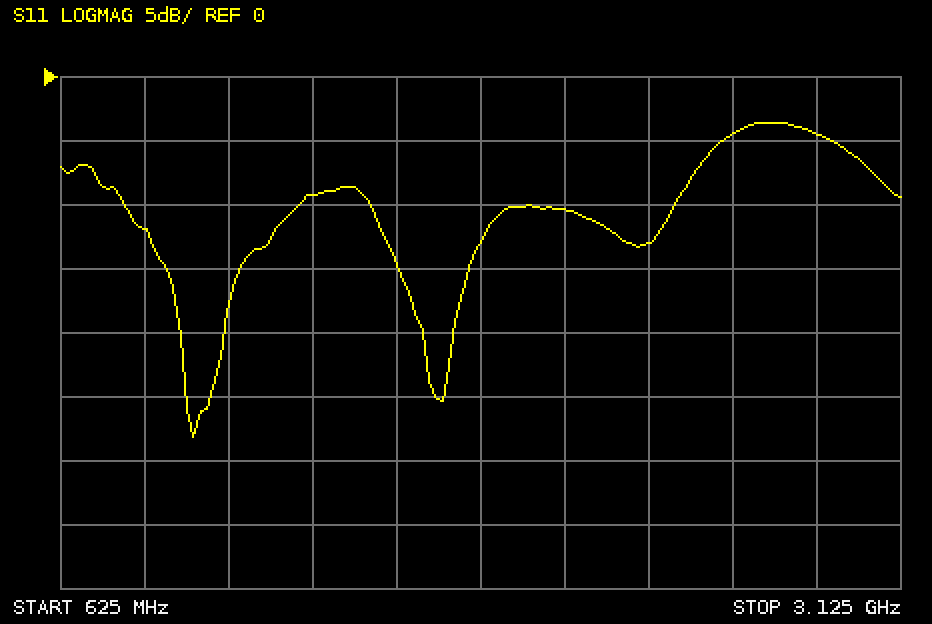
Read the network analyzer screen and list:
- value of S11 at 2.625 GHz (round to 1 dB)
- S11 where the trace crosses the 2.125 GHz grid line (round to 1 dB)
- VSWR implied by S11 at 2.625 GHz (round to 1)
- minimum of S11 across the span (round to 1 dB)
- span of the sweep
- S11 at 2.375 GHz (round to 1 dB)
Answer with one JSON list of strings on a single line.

["-4 dB", "-10 dB", "4", "-28 dB", "2.5 GHz", "-13 dB"]
